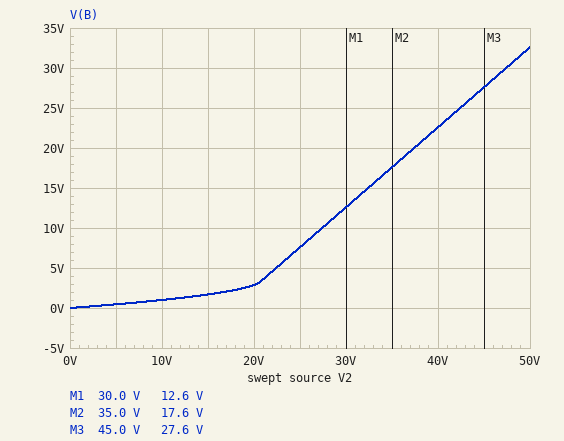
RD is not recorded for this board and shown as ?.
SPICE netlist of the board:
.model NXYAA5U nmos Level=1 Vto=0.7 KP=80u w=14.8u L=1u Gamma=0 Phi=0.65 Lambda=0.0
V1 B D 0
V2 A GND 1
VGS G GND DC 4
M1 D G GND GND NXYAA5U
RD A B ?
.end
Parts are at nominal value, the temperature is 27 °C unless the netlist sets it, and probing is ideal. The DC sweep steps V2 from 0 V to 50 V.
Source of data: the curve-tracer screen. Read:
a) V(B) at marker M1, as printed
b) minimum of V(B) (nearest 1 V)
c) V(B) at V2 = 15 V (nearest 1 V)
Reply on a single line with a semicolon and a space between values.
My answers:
12.6 V; 0 V; 2 V
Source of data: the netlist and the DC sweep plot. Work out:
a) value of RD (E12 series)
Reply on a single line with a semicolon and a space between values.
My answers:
2.7 kΩ
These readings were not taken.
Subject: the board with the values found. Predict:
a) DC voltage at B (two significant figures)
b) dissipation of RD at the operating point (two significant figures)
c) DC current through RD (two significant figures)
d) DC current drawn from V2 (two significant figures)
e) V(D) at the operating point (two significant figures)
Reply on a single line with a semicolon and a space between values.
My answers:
88 mV; 310 µW; 340 µA; 340 µA; 88 mV
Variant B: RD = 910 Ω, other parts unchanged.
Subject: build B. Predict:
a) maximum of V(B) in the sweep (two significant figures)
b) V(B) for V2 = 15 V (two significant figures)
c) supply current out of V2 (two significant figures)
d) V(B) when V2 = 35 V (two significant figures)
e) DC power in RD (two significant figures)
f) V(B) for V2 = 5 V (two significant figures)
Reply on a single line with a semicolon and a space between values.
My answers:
44 V; 9.1 V; 850 µA; 29 V; 660 µW; 1.3 V
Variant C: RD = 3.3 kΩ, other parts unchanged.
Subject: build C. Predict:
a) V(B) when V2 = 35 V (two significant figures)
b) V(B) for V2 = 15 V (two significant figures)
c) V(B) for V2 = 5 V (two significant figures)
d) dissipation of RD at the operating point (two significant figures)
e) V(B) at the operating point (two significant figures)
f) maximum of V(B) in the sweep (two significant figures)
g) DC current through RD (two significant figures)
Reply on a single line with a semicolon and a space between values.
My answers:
14 V; 1.3 V; 380 mV; 260 µW; 73 mV; 29 V; 280 µA
